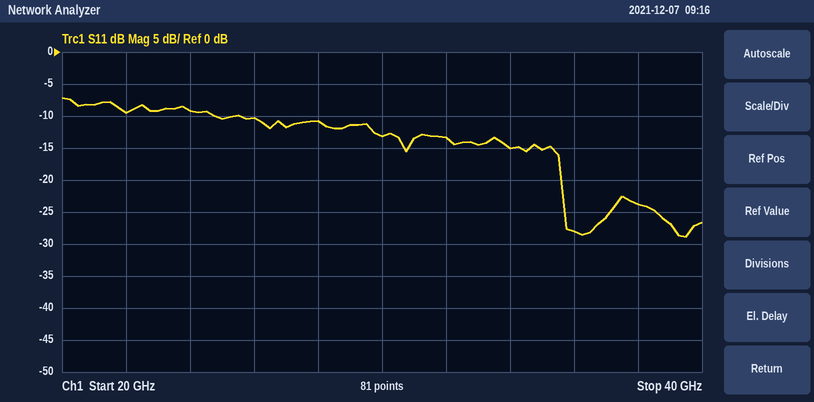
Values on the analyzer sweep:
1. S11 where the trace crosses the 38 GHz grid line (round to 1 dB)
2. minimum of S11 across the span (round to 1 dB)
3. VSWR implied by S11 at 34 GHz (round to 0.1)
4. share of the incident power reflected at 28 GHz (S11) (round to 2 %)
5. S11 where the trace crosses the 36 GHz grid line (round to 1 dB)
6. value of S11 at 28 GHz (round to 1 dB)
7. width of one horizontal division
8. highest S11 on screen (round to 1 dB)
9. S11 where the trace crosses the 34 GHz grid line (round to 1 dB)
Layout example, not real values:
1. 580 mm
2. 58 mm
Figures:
1. -24 dB
2. -29 dB
3. 1.4
4. 8 %
5. -28 dB
6. -11 dB
7. 2 GHz
8. -7 dB
9. -15 dB
